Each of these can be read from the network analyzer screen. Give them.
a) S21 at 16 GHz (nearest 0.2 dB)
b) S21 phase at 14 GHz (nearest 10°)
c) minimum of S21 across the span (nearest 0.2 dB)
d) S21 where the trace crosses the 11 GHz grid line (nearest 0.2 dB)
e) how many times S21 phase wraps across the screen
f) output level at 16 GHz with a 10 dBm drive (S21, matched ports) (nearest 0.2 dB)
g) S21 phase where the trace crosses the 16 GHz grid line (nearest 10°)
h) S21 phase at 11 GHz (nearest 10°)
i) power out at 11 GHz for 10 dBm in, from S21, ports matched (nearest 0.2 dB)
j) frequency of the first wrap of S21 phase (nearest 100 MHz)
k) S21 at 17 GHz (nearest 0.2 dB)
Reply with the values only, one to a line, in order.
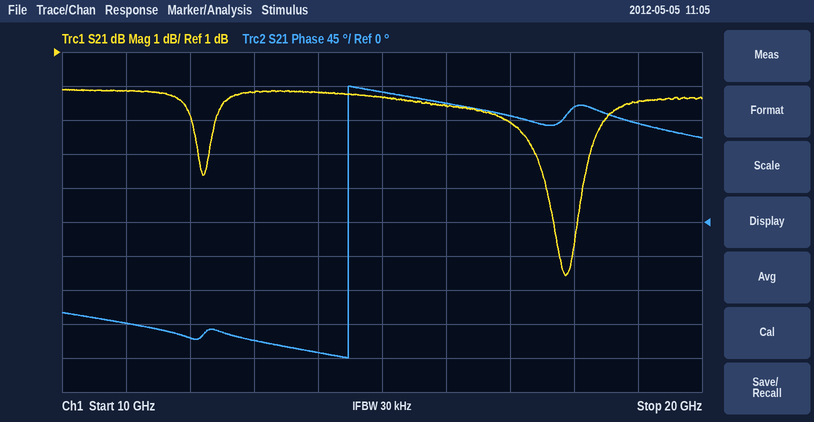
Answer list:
-0.6 dB
-170°
-5.6 dB
-0.2 dB
1
9.4 dBm
160°
-130°
9.8 dBm
14.5 GHz
-1.0 dB
